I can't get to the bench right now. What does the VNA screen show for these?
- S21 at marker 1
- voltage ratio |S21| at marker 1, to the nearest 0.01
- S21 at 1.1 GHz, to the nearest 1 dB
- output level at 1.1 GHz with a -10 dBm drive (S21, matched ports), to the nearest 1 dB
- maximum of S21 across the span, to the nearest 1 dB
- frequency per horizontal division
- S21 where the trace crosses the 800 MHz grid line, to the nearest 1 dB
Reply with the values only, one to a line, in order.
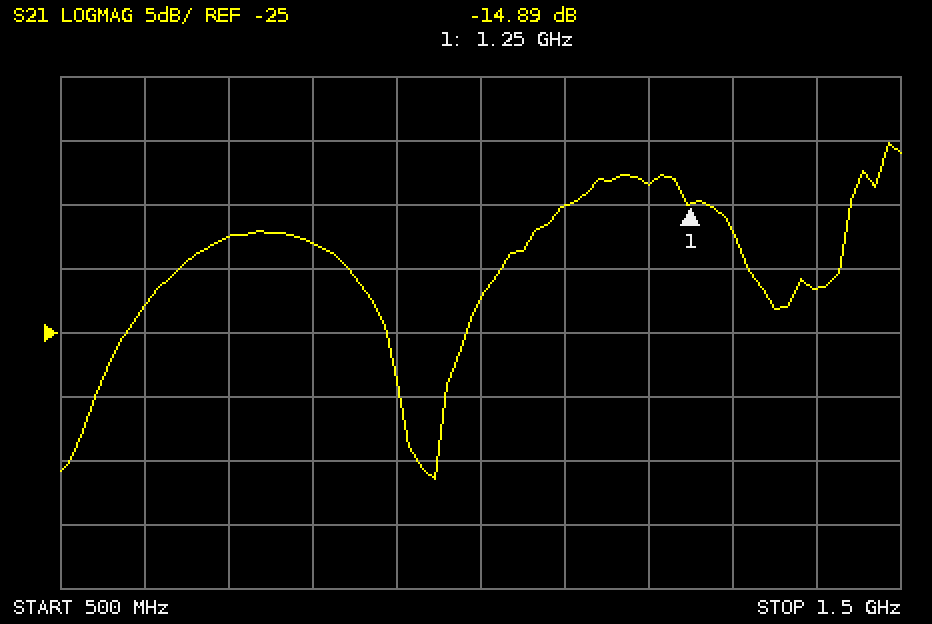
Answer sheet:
-14.89 dB
0.18
-15 dB
-25 dBm
-10 dB
100 MHz
-18 dB
